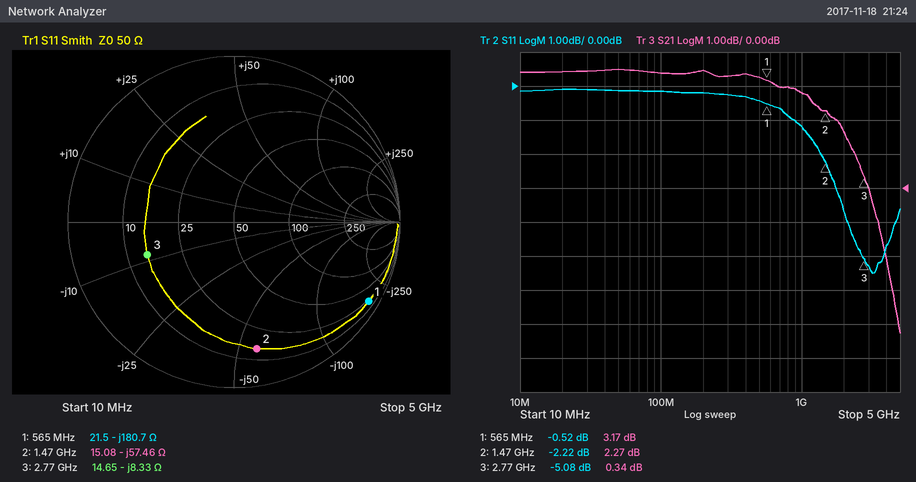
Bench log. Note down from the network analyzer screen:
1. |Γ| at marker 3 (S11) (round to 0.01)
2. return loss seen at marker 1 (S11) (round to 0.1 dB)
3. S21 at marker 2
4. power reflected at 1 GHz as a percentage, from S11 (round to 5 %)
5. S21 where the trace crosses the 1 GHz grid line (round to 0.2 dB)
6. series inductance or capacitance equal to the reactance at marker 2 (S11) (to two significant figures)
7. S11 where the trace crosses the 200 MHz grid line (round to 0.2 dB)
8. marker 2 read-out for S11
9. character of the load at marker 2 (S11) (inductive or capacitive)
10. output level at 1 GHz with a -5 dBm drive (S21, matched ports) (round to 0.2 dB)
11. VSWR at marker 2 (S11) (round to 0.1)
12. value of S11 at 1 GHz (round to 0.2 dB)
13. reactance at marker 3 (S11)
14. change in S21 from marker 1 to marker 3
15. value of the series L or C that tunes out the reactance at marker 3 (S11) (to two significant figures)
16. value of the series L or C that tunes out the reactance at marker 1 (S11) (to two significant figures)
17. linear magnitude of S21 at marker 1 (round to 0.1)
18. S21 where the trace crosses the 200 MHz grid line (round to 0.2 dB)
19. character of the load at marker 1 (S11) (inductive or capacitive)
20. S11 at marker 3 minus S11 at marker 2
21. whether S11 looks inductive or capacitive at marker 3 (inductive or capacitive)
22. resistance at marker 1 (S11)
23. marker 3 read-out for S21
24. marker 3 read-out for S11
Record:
0.56
0.5 dB
2.27 dB
75 %
2.8 dB
1.9 pF
-0.2 dB
-2.22 dB
capacitive
-2.2 dBm
7.9
-1.2 dB
-8.33 Ω
-2.83 dB
480 pH
51 nH
1.4
3.4 dB
capacitive
-2.86 dB
capacitive
21.5 Ω
0.34 dB
-5.08 dB
